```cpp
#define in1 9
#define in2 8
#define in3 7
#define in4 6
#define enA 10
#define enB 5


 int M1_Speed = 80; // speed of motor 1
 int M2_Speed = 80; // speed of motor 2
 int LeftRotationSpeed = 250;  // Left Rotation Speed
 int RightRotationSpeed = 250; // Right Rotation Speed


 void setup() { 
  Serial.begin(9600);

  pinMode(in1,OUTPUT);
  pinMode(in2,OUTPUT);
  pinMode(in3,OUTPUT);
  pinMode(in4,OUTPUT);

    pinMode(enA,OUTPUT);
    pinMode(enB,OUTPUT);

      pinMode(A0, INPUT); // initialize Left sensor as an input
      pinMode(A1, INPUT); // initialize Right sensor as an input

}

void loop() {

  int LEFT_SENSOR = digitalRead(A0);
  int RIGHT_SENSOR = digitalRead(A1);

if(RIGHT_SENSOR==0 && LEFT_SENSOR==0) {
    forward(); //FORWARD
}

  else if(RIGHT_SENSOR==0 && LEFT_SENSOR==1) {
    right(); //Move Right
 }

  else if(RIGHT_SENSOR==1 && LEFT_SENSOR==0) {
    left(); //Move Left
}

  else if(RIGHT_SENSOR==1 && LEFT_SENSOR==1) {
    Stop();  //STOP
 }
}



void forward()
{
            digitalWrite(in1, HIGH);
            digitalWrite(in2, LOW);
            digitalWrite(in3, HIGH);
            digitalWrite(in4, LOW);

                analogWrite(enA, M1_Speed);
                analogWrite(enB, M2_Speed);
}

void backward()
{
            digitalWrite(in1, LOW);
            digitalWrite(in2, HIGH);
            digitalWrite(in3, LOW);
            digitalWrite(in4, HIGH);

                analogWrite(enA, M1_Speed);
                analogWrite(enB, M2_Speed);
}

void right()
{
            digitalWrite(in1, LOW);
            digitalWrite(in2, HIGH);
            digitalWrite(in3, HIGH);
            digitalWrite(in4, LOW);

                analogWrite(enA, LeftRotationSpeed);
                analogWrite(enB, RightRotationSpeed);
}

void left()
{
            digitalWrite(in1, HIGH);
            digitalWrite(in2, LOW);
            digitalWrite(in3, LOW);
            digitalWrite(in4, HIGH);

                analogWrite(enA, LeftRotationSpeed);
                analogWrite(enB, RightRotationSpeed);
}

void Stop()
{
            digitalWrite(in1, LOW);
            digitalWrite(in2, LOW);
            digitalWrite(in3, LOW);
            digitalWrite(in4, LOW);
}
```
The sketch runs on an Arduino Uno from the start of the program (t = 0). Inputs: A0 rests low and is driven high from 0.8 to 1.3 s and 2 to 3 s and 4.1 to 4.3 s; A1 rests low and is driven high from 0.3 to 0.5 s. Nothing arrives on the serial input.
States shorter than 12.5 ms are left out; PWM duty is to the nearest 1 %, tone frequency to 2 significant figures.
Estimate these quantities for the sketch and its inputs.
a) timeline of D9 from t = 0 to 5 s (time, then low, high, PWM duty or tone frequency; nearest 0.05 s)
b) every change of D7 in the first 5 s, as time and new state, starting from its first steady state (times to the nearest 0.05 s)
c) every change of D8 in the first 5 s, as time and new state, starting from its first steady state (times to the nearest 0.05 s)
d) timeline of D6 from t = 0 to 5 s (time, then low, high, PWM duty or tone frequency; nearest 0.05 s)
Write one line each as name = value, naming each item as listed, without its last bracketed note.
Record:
timeline of D9 from t = 0 to 5 s = 0 s high; 0.8 s low; 1.3 s high; 2 s low; 3 s high; 4.1 s low; 4.3 s high
every change of D7 in the first 5 s, as time and new state, starting from its first steady state = 0 s high; 0.3 s low; 0.5 s high
every change of D8 in the first 5 s, as time and new state, starting from its first steady state = 0 s low; 0.8 s high; 1.3 s low; 2 s high; 3 s low; 4.1 s high; 4.3 s low
timeline of D6 from t = 0 to 5 s = 0 s low; 0.3 s high; 0.5 s low
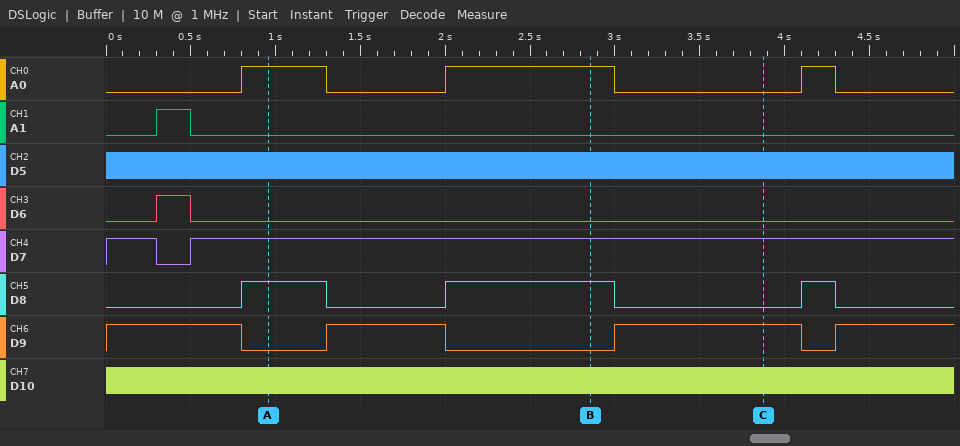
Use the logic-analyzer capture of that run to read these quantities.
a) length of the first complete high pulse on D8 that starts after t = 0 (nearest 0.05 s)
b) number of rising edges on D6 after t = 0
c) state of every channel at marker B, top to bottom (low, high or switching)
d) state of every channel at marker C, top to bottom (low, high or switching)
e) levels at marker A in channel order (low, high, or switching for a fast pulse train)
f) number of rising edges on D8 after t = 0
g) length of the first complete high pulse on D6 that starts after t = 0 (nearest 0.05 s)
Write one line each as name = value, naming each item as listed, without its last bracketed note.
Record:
length of the first complete high pulse on D8 that starts after t = 0 = 0.50 s
number of rising edges on D6 after t = 0 = 1
state of every channel at marker B, top to bottom = A0 high, A1 low, D5 switching, D6 low, D7 high, D8 high, D9 low, D10 switching
state of every channel at marker C, top to bottom = A0 low, A1 low, D5 switching, D6 low, D7 high, D8 low, D9 high, D10 switching
levels at marker A in channel order = A0 high, A1 low, D5 switching, D6 low, D7 high, D8 high, D9 low, D10 switching
number of rising edges on D8 after t = 0 = 3
length of the first complete high pulse on D6 that starts after t = 0 = 0.20 s
